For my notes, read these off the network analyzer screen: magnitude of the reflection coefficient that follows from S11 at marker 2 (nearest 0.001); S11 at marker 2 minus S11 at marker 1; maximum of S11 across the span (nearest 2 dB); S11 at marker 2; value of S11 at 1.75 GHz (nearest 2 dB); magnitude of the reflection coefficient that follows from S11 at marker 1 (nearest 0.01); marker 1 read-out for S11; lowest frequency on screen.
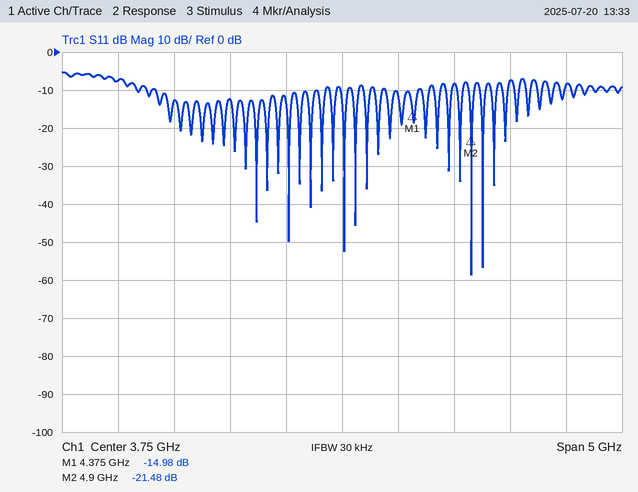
0.084
-6.50 dB
-6 dB
-21.48 dB
-8 dB
0.18
-14.98 dB
1.25 GHz
